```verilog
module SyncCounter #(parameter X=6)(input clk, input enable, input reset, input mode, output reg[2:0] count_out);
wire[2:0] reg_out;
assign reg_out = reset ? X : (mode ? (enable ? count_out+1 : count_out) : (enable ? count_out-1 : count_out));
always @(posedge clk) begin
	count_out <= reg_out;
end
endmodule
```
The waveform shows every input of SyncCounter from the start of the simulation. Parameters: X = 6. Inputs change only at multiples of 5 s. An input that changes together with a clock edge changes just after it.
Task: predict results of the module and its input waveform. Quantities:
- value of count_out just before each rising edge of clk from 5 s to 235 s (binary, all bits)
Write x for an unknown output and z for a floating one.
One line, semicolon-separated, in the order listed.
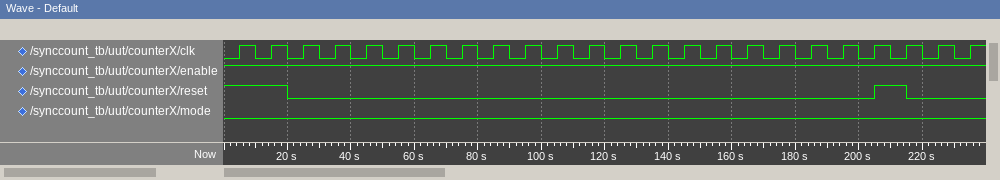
x, 110, 110, 101, 100, 011, 010, 001, 000, 111, 110, 101, 100, 011, 010, 001, 000, 111, 110, 101, 100, 011, 110, 101
